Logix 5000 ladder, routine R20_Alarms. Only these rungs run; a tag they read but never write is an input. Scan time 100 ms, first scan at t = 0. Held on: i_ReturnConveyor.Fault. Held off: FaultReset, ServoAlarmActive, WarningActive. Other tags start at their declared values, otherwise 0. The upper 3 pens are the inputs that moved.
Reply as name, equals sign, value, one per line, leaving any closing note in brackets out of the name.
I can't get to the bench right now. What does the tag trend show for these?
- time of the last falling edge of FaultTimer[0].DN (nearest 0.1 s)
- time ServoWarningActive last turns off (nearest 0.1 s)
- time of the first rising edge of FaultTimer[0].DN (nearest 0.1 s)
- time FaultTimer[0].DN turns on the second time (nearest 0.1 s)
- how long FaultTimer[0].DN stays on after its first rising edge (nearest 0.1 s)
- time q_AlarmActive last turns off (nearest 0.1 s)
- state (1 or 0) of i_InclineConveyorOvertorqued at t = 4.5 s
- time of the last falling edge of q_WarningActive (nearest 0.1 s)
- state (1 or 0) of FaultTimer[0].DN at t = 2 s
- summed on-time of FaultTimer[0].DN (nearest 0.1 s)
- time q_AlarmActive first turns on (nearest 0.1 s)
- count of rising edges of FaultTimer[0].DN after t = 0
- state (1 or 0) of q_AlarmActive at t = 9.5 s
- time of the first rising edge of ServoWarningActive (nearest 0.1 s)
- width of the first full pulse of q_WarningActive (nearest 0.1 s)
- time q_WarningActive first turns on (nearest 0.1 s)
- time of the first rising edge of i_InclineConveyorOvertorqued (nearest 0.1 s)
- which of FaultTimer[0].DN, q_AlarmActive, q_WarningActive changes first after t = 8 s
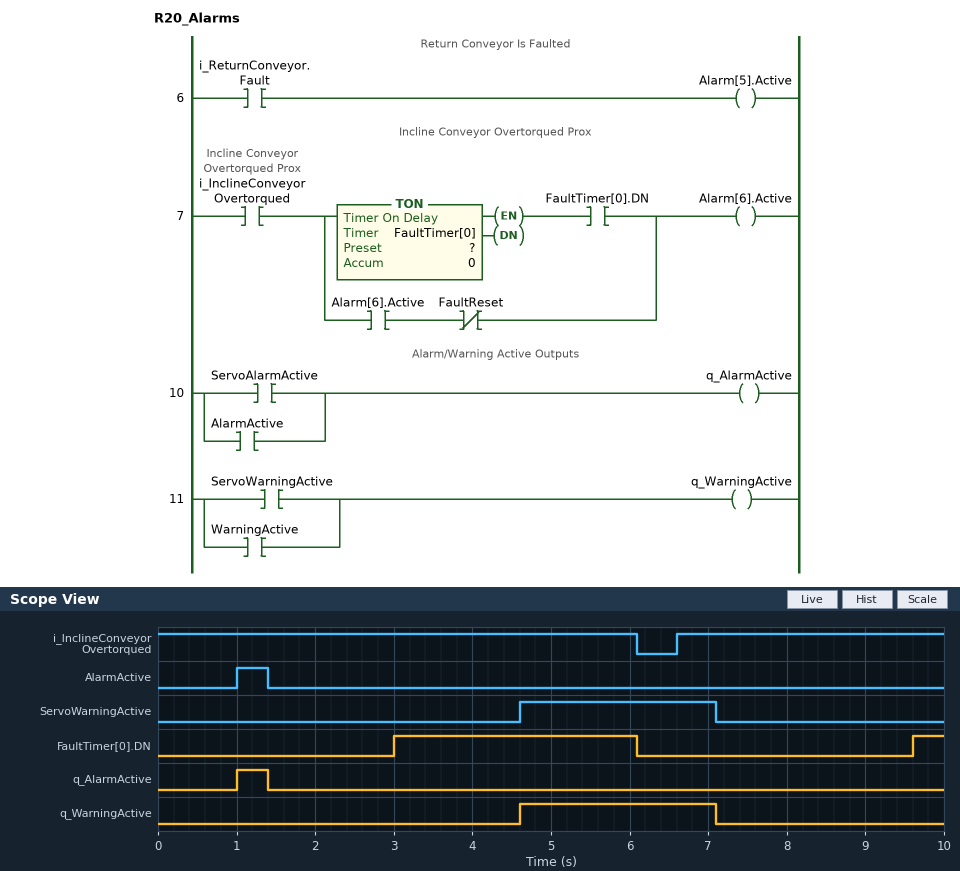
time of the last falling edge of FaultTimer[0].DN = 6.1 s
time ServoWarningActive last turns off = 7.1 s
time of the first rising edge of FaultTimer[0].DN = 3.0 s
time FaultTimer[0].DN turns on the second time = 9.6 s
how long FaultTimer[0].DN stays on after its first rising edge = 3.1 s
time q_AlarmActive last turns off = 1.4 s
state (1 or 0) of i_InclineConveyorOvertorqued at t = 4.5 s = 1
time of the last falling edge of q_WarningActive = 7.1 s
state (1 or 0) of FaultTimer[0].DN at t = 2 s = 0
summed on-time of FaultTimer[0].DN = 3.5 s
time q_AlarmActive first turns on = 1.0 s
count of rising edges of FaultTimer[0].DN after t = 0 = 2
state (1 or 0) of q_AlarmActive at t = 9.5 s = 0
time of the first rising edge of ServoWarningActive = 4.6 s
width of the first full pulse of q_WarningActive = 2.5 s
time q_WarningActive first turns on = 4.6 s
time of the first rising edge of i_InclineConveyorOvertorqued = 6.6 s
which of FaultTimer[0].DN, q_AlarmActive, q_WarningActive changes first after t = 8 s = FaultTimer[0].DN
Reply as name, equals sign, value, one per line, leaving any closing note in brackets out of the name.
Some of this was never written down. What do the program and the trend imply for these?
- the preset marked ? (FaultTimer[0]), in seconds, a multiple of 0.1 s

the preset marked ? (FaultTimer[0]), in seconds, a multiple of 0.1 s = 3.0 s
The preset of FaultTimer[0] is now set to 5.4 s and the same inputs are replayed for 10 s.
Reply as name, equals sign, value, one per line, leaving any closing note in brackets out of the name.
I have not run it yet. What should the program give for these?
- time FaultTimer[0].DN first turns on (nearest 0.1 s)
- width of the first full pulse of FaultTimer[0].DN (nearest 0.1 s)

time FaultTimer[0].DN first turns on = 5.4 s
width of the first full pulse of FaultTimer[0].DN = 0.7 s
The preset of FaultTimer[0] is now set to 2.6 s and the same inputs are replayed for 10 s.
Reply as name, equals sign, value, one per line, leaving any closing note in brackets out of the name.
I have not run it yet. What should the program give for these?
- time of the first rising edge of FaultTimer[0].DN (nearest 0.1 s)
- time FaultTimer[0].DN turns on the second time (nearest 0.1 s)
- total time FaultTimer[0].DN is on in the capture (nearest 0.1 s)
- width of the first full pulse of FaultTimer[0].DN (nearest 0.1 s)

time of the first rising edge of FaultTimer[0].DN = 2.6 s
time FaultTimer[0].DN turns on the second time = 9.2 s
total time FaultTimer[0].DN is on in the capture = 4.3 s
width of the first full pulse of FaultTimer[0].DN = 3.5 s
